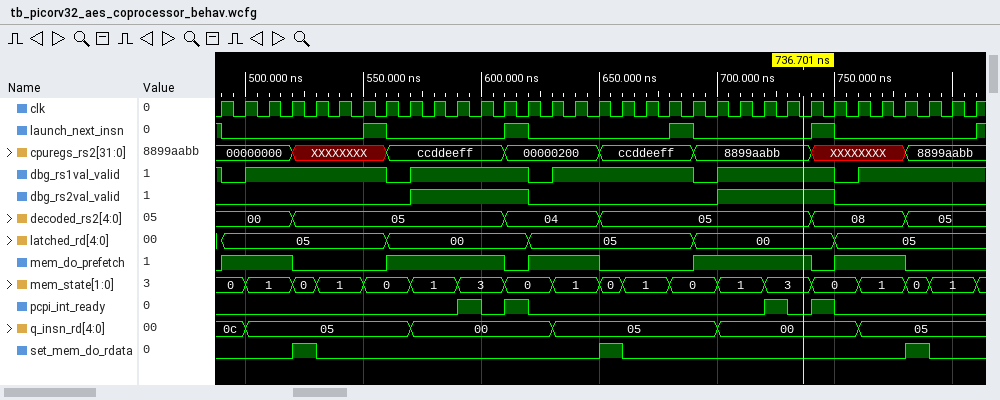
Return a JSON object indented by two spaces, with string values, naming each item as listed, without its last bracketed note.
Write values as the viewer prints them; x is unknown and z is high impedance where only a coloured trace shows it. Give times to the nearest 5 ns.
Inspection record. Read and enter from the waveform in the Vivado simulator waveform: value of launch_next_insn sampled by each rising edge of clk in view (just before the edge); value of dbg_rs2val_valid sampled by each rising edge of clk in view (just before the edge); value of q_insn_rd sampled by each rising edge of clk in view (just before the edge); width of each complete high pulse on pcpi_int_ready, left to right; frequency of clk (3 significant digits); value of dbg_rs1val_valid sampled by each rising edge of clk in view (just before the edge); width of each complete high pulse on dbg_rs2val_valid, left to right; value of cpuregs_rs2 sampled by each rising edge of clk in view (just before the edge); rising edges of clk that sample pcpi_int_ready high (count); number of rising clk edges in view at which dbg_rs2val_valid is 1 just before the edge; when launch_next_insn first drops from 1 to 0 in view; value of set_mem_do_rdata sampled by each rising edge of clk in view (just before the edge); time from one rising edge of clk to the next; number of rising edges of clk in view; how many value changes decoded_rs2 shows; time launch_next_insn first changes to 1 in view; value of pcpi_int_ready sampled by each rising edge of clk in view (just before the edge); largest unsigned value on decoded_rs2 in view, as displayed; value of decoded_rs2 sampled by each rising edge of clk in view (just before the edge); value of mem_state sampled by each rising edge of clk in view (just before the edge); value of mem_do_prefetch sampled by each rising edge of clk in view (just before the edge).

{
  "value of launch_next_insn sampled by each rising edge of clk in view": "1 0 0 0 0 0 0 1 0 0 0 0 0 1 0 0 0 0 0 0 1 0 0 0 0 0 1 0 0 0 0 0 0",
  "value of dbg_rs2val_valid sampled by each rising edge of clk in view": "0 0 0 0 0 0 0 0 0 1 1 1 1 1 0 0 0 0 0 0 0 0 1 1 1 1 1 0 0 0 0 0 0",
  "value of q_insn_rd sampled by each rising edge of clk in view": "0c, 0c, 05, 05, 05, 05, 05, 05, 05, 00, 00, 00, 00, 00, 00, 05, 05, 05, 05, 05, 05, 05, 00, 00, 00, 00, 00, 00, 05, 05, 05, 05, 05",
  "width of each complete high pulse on pcpi_int_ready, left to right": "10 ns, 10 ns, 10 ns, 10 ns",
  "frequency of clk": "100 MHz",
  "value of dbg_rs1val_valid sampled by each rising edge of clk in view": "1 0 1 1 1 1 1 1 0 1 1 1 1 1 0 1 1 1 1 1 1 0 1 1 1 1 1 0 1 1 1 1 1",
  "width of each complete high pulse on dbg_rs2val_valid, left to right": "50 ns, 50 ns",
  "value of cpuregs_rs2 sampled by each rising edge of clk in view": "00000000, 00000000, 00000000, 00000000, XXXXXXXX, XXXXXXXX, XXXXXXXX, XXXXXXXX, ccddeeff, ccddeeff, ccddeeff, ccddeeff, ccddeeff, 00000200, 00000200, 00000200, 00000200, ccddeeff, ccddeeff, ccddeeff, ccddeeff, 8899aabb, 8899aabb, 8899aabb, 8899aabb, 8899aabb, XXXXXXXX, XXXXXXXX, XXXXXXXX, XXXXXXXX, 8899aabb, 8899aabb, 8899aabb",
  "rising edges of clk that sample pcpi_int_ready high": "4",
  "number of rising clk edges in view at which dbg_rs2val_valid is 1 just before the edge": "10",
  "when launch_next_insn first drops from 1 to 0 in view": "490 ns",
  "value of set_mem_do_rdata sampled by each rising edge of clk in view": "0 0 0 0 1 0 0 0 0 0 0 0 0 0 0 0 0 1 0 0 0 0 0 0 0 0 0 0 0 0 1 0 0",
  "time from one rising edge of clk to the next": "10 ns",
  "number of rising edges of clk in view": "33",
  "how many value changes decoded_rs2 shows": "5",
  "time launch_next_insn first changes to 1 in view": "550 ns",
  "value of pcpi_int_ready sampled by each rising edge of clk in view": "0 0 0 0 0 0 0 0 0 0 0 1 0 1 0 0 0 0 0 0 0 0 0 0 1 0 1 0 0 0 0 0 0",
  "largest unsigned value on decoded_rs2 in view, as displayed": "08",
  "value of decoded_rs2 sampled by each rising edge of clk in view": "00, 00, 00, 00, 05, 05, 05, 05, 05, 05, 05, 05, 05, 04, 04, 04, 04, 05, 05, 05, 05, 05, 05, 05, 05, 05, 08, 08, 08, 08, 05, 05, 05",
  "value of mem_state sampled by each rising edge of clk in view": "0, 0, 1, 1, 0, 1, 1, 0, 0, 1, 1, 3, 3, 0, 0, 1, 1, 0, 1, 1, 0, 0, 1, 1, 3, 3, 0, 0, 1, 1, 0, 1, 1",
  "value of mem_do_prefetch sampled by each rising edge of clk in view": "0 1 1 1 0 0 0 0 1 1 1 1 1 0 1 1 1 0 0 0 0 1 1 1 1 1 0 1 1 1 0 0 0"
}
